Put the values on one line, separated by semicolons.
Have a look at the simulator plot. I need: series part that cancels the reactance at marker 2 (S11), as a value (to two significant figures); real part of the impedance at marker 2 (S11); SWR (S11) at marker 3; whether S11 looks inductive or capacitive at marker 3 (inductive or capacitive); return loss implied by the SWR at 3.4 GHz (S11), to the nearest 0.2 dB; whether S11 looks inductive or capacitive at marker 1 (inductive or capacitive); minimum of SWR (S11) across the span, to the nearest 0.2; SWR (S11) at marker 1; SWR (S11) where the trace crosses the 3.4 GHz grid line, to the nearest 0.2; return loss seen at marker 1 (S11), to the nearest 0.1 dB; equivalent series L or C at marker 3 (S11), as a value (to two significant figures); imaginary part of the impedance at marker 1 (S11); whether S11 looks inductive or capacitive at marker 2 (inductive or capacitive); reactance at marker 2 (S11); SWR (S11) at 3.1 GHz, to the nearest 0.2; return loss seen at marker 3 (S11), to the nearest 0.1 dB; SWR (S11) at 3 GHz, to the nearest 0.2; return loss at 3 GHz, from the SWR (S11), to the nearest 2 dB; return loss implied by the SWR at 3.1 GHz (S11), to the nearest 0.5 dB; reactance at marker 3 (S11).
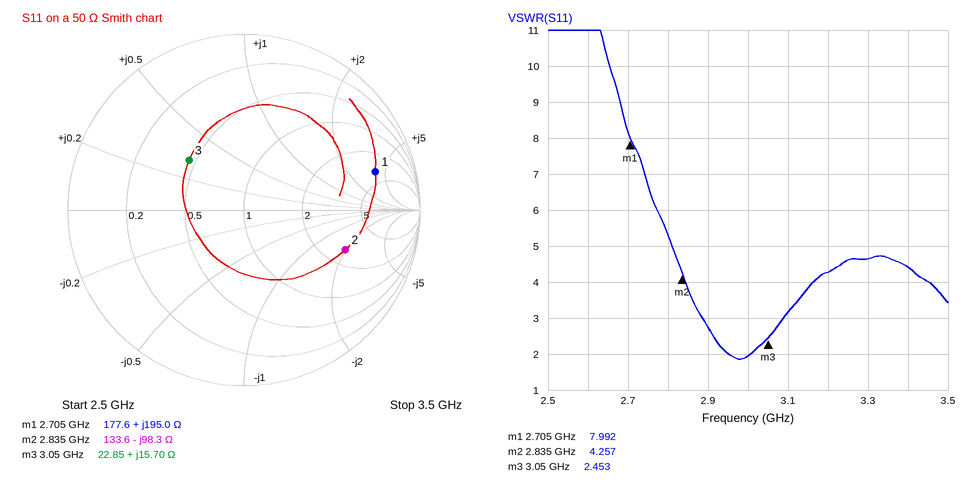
5.5 nH; 133.6 Ω; 2.453; inductive; 4.0 dB; inductive; 1.8; 7.992; 4.4; 2.2 dB; 820 pH; +195.0 Ω; capacitive; -98.3 Ω; 3.2; 7.5 dB; 2.0; 10 dB; 5.5 dB; +15.70 Ω
